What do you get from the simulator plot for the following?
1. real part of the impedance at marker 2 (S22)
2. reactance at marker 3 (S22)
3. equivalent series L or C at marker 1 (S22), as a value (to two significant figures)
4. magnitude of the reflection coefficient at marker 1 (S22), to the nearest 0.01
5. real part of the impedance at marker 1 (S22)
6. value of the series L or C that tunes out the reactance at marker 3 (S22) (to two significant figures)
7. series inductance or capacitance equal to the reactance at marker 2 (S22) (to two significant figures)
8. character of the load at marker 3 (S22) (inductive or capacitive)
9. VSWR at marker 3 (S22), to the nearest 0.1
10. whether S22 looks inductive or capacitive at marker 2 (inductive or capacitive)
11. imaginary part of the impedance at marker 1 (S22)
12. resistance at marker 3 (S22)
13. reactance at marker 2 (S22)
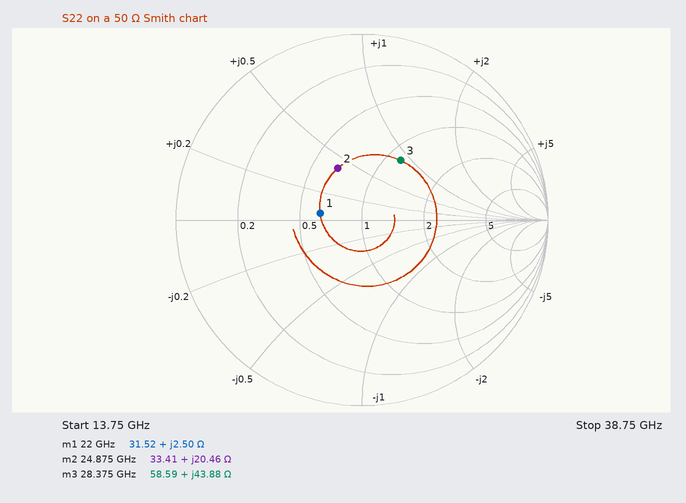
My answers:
33.41 Ω
+43.88 Ω
18 pH
0.23
31.52 Ω
130 fF
130 pH
inductive
2.2
inductive
+2.50 Ω
58.59 Ω
+20.46 Ω
